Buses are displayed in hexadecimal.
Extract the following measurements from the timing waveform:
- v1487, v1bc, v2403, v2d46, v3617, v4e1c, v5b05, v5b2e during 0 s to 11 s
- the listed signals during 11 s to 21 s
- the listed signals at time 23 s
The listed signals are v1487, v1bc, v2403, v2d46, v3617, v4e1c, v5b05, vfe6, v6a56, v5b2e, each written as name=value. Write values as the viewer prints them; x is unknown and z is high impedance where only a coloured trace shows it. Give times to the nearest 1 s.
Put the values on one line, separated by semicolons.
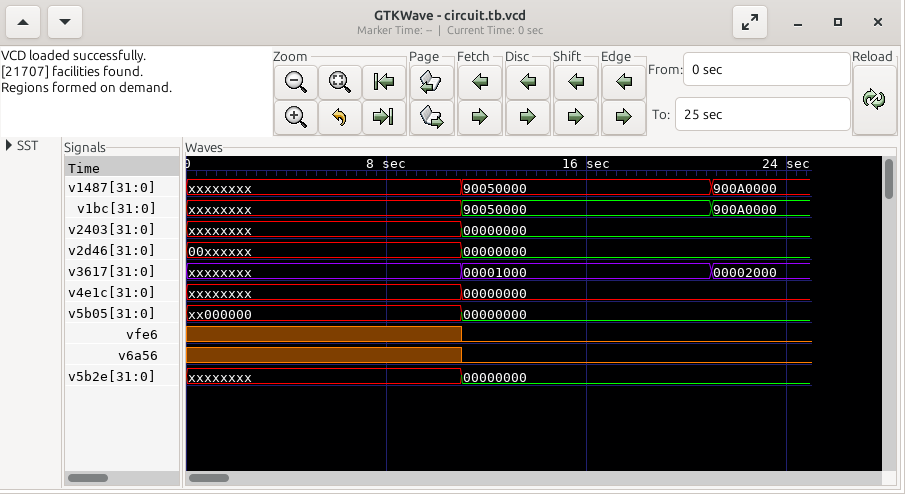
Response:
v1487=xxxxxxxx, v1bc=xxxxxxxx, v2403=xxxxxxxx, v2d46=00xxxxxx, v3617=xxxxxxxx, v4e1c=xxxxxxxx, v5b05=xx000000, v5b2e=xxxxxxxx; v1487=90050000, v1bc=90050000, v2403=00000000, v2d46=00000000, v3617=00001000, v4e1c=00000000, v5b05=00000000, vfe6=0, v6a56=0, v5b2e=00000000; v1487=900A0000, v1bc=900A0000, v2403=00000000, v2d46=00000000, v3617=00002000, v4e1c=00000000, v5b05=00000000, vfe6=0, v6a56=0, v5b2e=00000000
